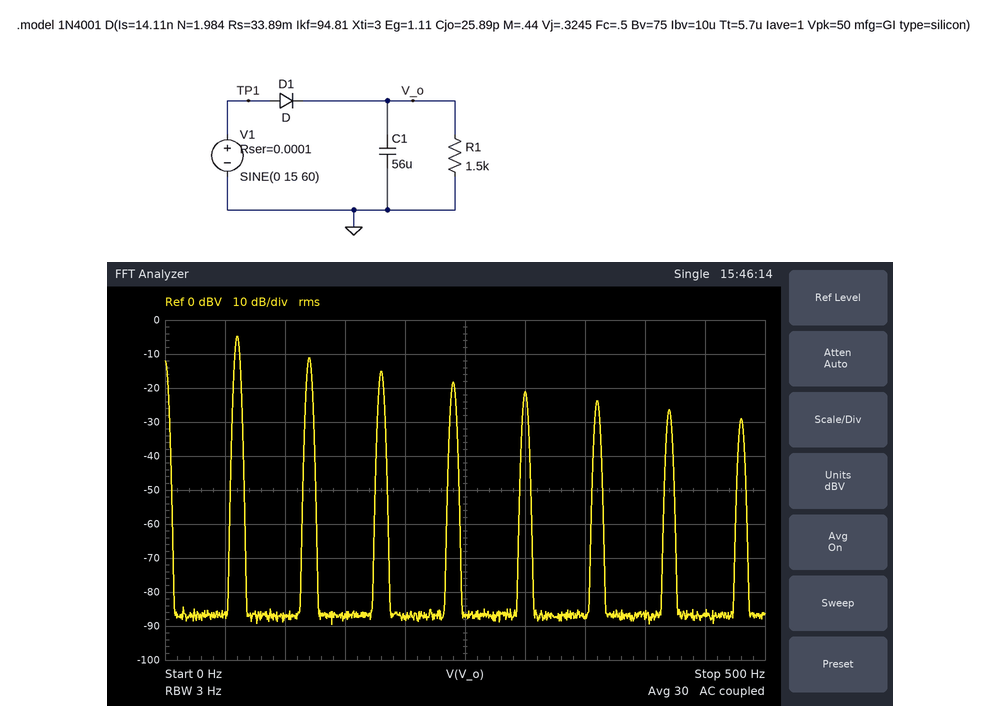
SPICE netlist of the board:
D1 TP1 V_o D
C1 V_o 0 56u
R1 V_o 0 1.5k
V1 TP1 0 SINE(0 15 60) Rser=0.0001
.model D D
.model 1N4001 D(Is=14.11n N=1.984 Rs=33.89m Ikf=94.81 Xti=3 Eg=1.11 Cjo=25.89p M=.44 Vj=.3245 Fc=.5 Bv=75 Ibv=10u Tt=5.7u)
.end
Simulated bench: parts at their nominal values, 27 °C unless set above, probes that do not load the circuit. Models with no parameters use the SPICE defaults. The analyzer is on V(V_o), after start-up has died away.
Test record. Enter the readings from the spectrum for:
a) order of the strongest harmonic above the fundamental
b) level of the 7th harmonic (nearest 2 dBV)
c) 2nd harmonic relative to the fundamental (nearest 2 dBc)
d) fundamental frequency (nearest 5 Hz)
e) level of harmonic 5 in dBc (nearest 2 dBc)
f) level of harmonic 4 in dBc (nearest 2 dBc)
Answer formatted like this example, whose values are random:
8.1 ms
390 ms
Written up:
2
-26 dBV
-6 dBc
60 Hz
-16 dBc
-14 dBc
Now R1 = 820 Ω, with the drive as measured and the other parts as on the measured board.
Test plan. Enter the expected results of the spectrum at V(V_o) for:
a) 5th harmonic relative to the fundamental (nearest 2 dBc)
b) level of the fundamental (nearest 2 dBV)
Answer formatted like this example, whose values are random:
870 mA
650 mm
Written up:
-18 dBc
0 dBV
